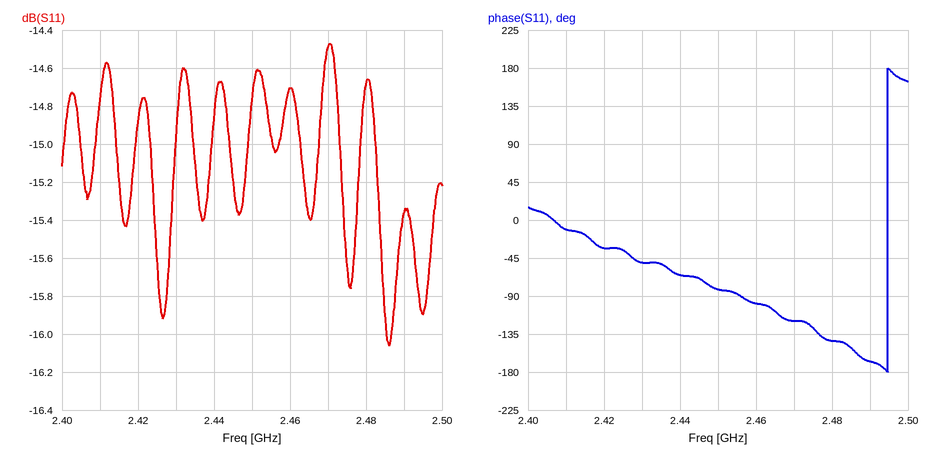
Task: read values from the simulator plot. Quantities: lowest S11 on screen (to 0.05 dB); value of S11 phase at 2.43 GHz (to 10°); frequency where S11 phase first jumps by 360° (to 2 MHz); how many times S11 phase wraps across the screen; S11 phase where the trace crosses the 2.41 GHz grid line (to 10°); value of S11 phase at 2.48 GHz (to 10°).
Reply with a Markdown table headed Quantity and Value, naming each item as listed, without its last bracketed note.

| Quantity | Value |
|---|---|
| lowest S11 on screen | -16.05 dB |
| value of S11 phase at 2.43 GHz | -50° |
| frequency where S11 phase first jumps by 360° | 2.494 GHz |
| how many times S11 phase wraps across the screen | 1 |
| S11 phase where the trace crosses the 2.41 GHz grid line | -10° |
| value of S11 phase at 2.48 GHz | -140° |
